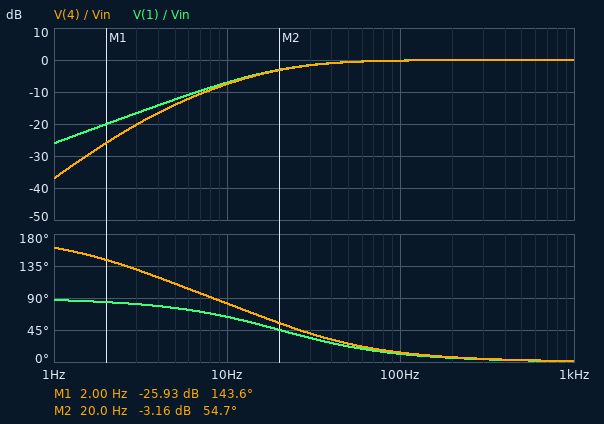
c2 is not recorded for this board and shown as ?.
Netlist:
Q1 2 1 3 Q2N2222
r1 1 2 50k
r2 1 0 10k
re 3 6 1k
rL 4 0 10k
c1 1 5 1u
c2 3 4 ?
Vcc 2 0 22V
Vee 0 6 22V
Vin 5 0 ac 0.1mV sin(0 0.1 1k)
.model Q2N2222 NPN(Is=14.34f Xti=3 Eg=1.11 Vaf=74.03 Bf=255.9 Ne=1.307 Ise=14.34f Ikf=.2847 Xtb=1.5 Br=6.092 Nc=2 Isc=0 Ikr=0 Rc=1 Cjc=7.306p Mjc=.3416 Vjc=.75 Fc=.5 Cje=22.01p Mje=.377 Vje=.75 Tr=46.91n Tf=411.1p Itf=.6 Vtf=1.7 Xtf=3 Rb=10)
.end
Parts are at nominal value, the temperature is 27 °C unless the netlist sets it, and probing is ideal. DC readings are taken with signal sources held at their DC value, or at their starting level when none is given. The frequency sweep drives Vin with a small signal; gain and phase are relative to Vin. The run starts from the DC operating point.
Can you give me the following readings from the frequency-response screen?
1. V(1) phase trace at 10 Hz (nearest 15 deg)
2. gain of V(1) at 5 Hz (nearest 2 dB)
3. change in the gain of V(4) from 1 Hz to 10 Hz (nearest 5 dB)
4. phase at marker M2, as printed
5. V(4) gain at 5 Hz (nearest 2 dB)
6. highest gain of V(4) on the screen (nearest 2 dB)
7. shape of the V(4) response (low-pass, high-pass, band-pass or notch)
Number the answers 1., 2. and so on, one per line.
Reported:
1. 60 deg
2. -12 dB
3. 30 dB
4. 54.7 deg
5. -14 dB
6. 0 dB
7. high-pass
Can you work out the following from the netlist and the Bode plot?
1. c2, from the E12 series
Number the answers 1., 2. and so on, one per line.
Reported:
1. 4.7 µF
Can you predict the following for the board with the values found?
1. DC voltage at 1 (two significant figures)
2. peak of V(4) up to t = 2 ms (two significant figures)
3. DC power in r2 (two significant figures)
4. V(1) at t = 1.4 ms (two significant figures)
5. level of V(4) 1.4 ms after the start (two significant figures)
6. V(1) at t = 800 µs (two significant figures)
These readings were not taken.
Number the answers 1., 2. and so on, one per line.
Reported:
1. 2.8 V
2. 98 mV
3. 770 µW
4. 2.8 V
5. 55 mV
6. 2.7 V
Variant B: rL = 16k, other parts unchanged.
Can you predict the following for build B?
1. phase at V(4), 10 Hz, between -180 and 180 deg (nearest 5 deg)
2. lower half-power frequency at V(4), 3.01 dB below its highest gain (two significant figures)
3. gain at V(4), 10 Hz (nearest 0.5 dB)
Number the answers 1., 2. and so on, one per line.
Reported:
1. 75 deg
2. 20 Hz
3. -7.0 dB
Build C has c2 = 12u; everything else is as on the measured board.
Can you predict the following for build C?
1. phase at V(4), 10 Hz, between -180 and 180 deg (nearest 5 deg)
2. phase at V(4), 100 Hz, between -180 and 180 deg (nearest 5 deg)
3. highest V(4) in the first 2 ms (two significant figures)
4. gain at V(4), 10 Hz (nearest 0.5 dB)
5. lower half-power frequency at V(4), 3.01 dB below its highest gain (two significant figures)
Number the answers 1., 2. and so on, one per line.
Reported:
1. 70 deg
2. 10 deg
3. 98 mV
4. -7.0 dB
5. 20 Hz
